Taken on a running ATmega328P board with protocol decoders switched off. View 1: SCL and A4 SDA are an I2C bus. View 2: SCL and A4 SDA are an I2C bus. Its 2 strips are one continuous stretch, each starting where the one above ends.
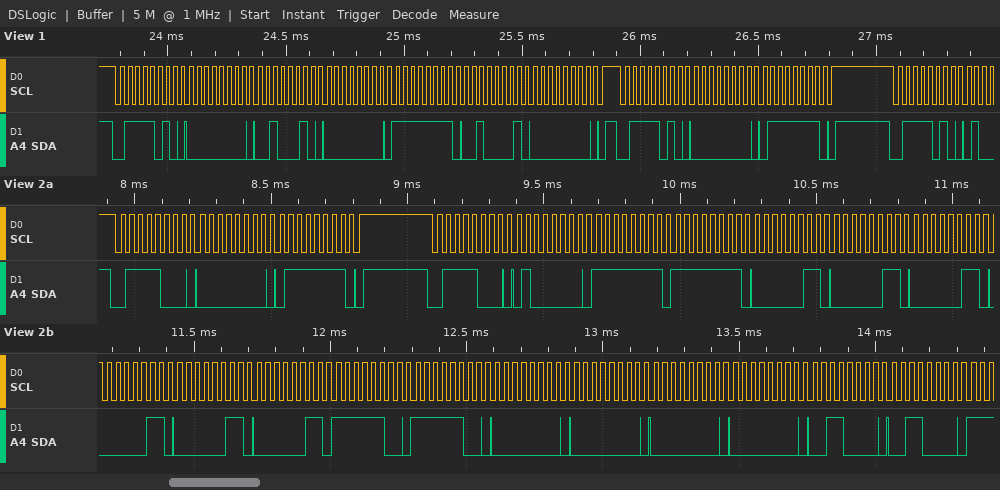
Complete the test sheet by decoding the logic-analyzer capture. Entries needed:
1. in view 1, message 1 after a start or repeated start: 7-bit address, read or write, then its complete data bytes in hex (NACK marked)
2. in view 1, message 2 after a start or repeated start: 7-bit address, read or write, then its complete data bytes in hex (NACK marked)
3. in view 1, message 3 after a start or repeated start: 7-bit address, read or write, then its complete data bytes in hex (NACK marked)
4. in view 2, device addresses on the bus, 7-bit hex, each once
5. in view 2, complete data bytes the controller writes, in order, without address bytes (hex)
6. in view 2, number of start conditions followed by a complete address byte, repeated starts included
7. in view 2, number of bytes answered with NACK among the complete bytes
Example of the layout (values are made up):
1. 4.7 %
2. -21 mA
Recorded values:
1. 0x3D write: 00 22 00 FF 21 00
2. 0x3D write: 00 7F
3. 0x3D write
4. 0x3C
5. 00 7F 40 FF FF 03 03 03 03 03 03 FC FC 00 00 00 00 30 30
6. 2
7. 0
